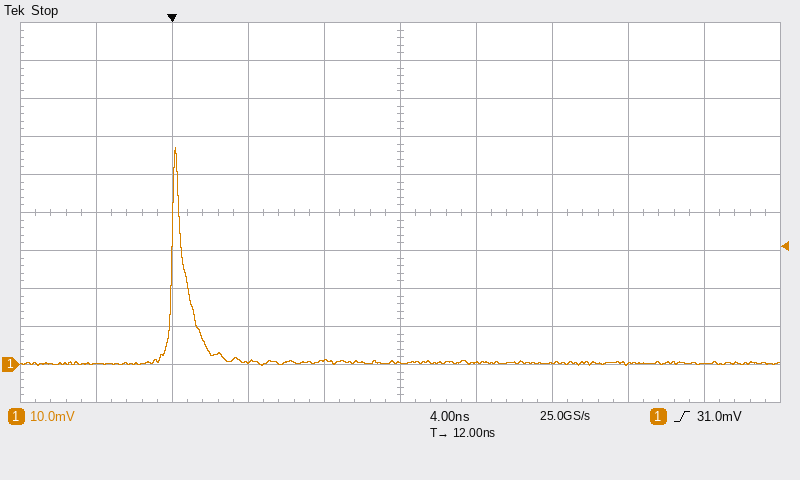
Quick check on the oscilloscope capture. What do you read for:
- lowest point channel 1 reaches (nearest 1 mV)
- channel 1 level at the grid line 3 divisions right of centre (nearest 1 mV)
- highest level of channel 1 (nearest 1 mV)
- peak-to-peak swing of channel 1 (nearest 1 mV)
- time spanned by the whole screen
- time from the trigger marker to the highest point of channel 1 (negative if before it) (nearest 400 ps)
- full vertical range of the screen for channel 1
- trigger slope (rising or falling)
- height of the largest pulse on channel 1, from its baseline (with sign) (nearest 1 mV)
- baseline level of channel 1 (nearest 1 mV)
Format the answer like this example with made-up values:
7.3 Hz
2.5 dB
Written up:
0 mV
0 mV
57 mV
57 mV
40 ns
0.0 ns
100 mV
rising
+57 mV
0 mV
